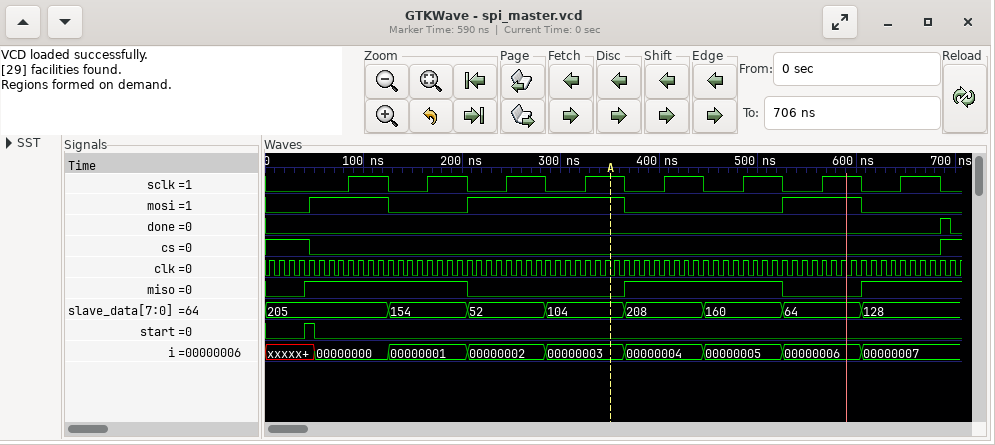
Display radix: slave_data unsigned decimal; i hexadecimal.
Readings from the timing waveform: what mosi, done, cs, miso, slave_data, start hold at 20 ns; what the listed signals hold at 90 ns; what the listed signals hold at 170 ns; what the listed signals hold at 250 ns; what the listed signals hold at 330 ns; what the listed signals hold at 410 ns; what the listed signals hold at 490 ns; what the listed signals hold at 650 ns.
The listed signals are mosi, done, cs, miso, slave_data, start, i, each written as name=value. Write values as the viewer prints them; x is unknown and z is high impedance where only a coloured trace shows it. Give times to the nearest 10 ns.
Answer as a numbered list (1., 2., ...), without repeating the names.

1. mosi=0, done=0, cs=1, miso=0, slave_data=205, start=0
2. mosi=1, done=0, cs=0, miso=1, slave_data=205, start=0, i=00000000
3. mosi=0, done=0, cs=0, miso=1, slave_data=154, start=0, i=00000001
4. mosi=1, done=0, cs=0, miso=0, slave_data=52, start=0, i=00000002
5. mosi=1, done=0, cs=0, miso=0, slave_data=104, start=0, i=00000003
6. mosi=0, done=0, cs=0, miso=1, slave_data=208, start=0, i=00000004
7. mosi=0, done=0, cs=0, miso=1, slave_data=160, start=0, i=00000005
8. mosi=0, done=0, cs=0, miso=1, slave_data=128, start=0, i=00000007
